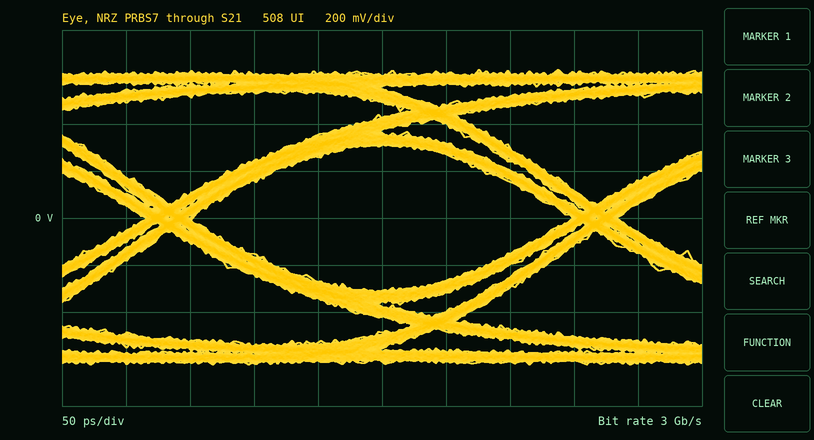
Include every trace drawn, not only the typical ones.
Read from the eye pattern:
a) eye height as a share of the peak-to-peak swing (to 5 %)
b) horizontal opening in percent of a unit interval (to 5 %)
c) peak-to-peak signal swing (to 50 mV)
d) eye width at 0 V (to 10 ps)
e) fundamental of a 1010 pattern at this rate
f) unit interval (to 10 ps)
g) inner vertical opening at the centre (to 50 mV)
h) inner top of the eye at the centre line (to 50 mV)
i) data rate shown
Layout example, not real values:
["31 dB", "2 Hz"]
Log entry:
["50 %", "90 %", "1.25 V", "300 ps", "1.5 GHz", "330 ps", "600 mV", "300 mV", "3 Gb/s"]
